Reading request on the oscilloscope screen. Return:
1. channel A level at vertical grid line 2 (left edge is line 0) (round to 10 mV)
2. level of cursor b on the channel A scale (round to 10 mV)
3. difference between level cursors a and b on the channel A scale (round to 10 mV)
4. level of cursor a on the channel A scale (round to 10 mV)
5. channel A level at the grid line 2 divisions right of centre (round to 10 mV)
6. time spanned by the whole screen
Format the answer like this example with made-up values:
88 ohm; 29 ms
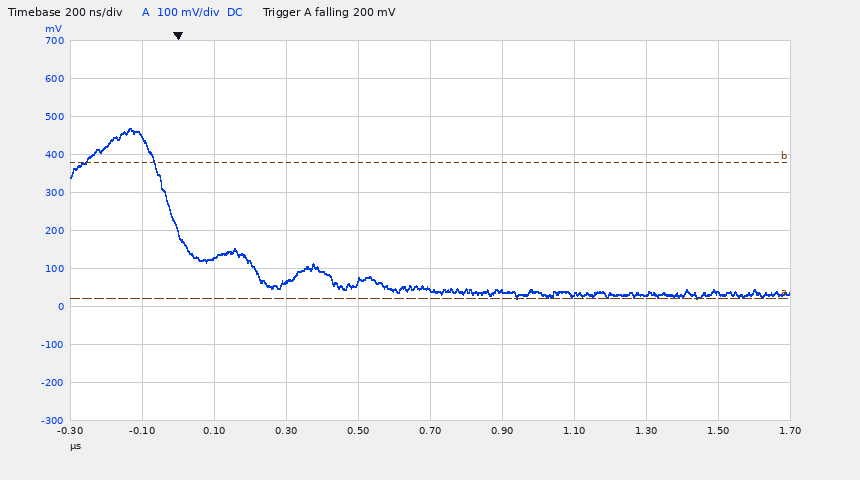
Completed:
130 mV; 380 mV; 360 mV; 20 mV; 30 mV; 2 µs
